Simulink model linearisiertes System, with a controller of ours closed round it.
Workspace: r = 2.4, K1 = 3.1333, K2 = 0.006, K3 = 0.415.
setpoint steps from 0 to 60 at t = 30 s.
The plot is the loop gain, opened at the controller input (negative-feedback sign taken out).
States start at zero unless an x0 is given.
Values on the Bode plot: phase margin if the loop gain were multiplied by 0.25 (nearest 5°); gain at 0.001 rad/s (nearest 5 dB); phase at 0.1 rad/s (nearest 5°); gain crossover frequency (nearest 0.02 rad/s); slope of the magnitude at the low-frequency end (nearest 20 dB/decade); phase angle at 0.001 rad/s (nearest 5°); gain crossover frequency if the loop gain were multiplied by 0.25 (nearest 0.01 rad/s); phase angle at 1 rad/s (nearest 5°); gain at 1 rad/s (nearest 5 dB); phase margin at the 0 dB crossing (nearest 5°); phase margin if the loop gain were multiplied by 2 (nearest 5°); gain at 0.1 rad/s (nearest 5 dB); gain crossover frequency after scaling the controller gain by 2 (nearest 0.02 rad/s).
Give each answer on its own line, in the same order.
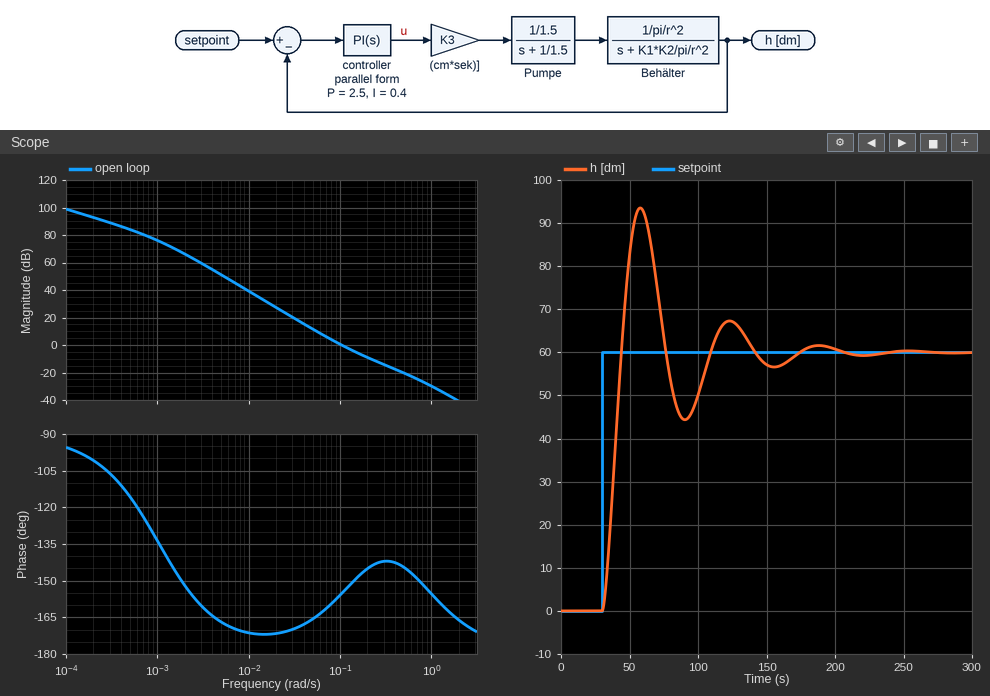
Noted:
15°
75 dB
-155°
0.10 rad/s
-20 dB/decade
-135°
0.05 rad/s
-155°
-30 dB
25°
30°
0 dB
0.16 rad/s
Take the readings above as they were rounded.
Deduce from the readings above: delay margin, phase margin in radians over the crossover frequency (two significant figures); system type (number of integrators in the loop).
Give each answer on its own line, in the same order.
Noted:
4.4 s
1
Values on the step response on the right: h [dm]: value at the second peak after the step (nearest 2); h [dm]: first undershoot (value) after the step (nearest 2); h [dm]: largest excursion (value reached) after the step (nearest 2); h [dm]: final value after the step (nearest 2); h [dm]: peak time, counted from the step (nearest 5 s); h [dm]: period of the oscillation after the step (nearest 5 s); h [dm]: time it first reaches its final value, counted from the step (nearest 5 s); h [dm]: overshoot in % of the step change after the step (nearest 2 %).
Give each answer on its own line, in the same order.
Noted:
68
44
94
60
30 s
65 s
15 s
56 %
